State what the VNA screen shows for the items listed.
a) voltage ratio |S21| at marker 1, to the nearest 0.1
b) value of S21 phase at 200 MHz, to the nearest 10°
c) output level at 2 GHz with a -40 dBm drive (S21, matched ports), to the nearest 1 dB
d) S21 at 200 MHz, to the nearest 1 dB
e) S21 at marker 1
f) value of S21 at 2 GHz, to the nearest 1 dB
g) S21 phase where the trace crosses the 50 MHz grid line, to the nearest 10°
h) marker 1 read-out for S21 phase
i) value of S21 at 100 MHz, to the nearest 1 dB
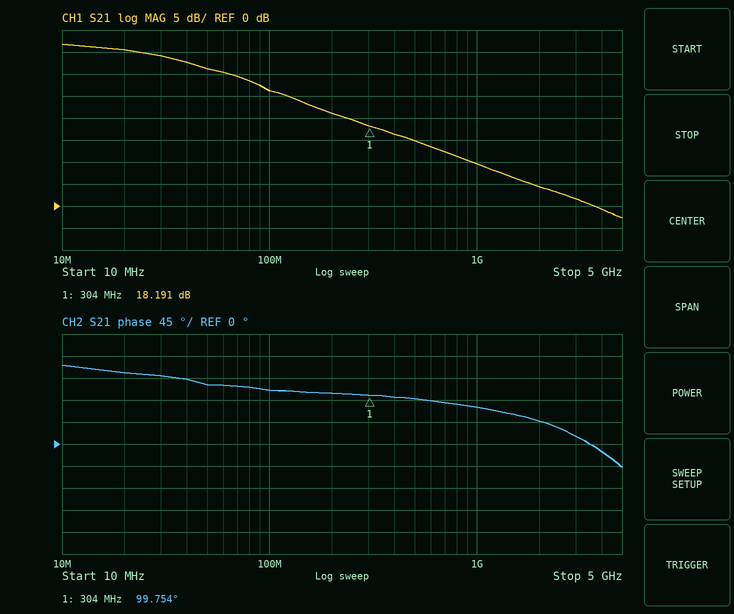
8.1
100°
-36 dBm
21 dB
18.191 dB
4 dB
120°
99.754°
26 dB
